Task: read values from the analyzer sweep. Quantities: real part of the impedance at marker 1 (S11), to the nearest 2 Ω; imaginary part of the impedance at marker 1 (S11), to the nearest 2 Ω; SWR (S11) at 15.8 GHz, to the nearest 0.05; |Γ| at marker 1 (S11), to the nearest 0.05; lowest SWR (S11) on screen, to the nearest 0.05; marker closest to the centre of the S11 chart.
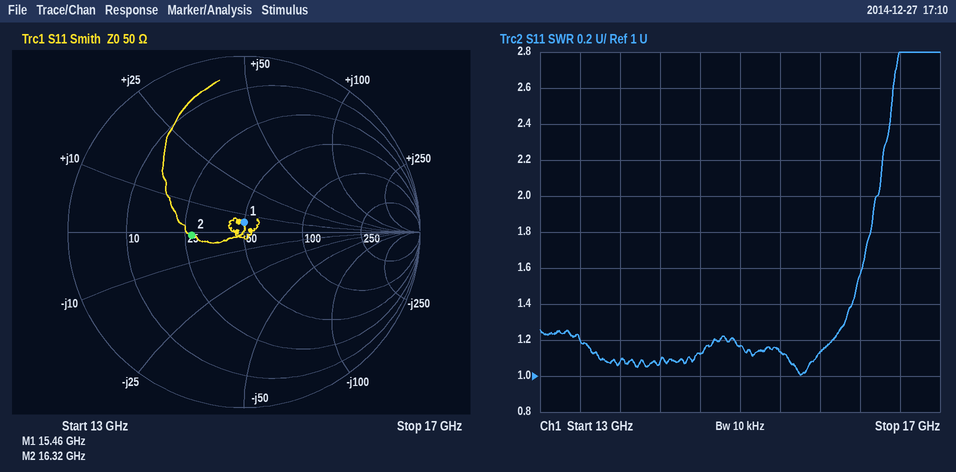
50 Ω
+6 Ω
1.15
0.05
1.00
marker 1
